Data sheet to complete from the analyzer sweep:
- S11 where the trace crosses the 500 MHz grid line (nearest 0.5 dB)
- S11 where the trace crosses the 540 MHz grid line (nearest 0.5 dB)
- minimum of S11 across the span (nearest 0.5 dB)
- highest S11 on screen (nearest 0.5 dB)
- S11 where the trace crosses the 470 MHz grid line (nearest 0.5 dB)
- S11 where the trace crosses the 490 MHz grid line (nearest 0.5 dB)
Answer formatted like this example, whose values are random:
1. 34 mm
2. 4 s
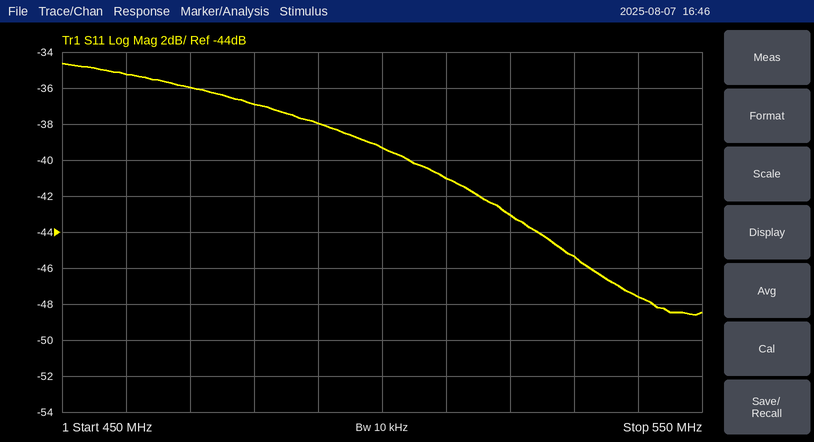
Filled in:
1. -39.5 dB
2. -47.5 dB
3. -48.5 dB
4. -34.5 dB
5. -36.0 dB
6. -38.0 dB
